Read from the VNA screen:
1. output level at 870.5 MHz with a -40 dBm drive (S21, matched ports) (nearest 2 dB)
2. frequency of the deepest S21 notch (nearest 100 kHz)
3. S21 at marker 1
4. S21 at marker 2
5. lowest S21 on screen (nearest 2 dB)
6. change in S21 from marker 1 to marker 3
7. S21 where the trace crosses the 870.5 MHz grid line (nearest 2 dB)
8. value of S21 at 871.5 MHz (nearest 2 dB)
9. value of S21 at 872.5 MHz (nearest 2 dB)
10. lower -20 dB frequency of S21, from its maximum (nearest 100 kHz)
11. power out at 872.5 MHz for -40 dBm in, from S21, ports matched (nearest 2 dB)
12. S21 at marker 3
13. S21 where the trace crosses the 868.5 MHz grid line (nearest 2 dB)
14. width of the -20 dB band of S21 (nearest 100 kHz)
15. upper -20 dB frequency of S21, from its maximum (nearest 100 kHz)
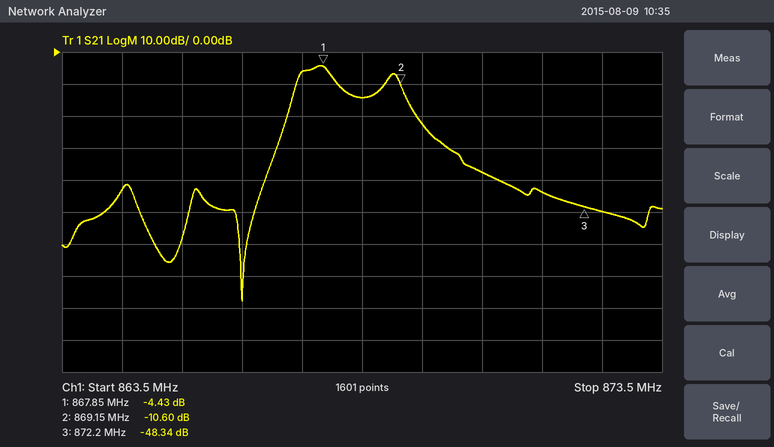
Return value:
-78 dBm
866.5 MHz
-4.43 dB
-10.60 dB
-78 dB
-43.91 dB
-38 dB
-44 dB
-50 dB
867.2 MHz
-90 dBm
-48.34 dB
-14 dB
2.4 MHz
869.6 MHz
